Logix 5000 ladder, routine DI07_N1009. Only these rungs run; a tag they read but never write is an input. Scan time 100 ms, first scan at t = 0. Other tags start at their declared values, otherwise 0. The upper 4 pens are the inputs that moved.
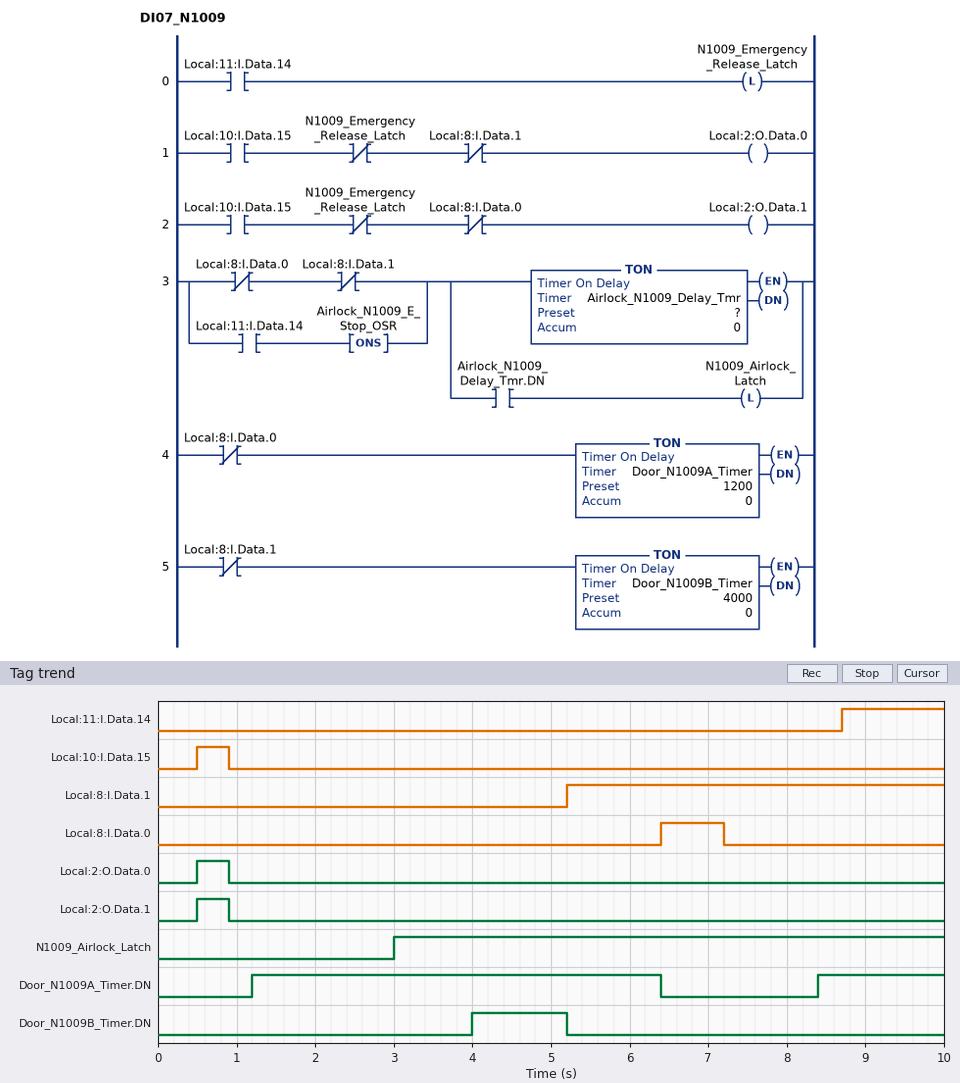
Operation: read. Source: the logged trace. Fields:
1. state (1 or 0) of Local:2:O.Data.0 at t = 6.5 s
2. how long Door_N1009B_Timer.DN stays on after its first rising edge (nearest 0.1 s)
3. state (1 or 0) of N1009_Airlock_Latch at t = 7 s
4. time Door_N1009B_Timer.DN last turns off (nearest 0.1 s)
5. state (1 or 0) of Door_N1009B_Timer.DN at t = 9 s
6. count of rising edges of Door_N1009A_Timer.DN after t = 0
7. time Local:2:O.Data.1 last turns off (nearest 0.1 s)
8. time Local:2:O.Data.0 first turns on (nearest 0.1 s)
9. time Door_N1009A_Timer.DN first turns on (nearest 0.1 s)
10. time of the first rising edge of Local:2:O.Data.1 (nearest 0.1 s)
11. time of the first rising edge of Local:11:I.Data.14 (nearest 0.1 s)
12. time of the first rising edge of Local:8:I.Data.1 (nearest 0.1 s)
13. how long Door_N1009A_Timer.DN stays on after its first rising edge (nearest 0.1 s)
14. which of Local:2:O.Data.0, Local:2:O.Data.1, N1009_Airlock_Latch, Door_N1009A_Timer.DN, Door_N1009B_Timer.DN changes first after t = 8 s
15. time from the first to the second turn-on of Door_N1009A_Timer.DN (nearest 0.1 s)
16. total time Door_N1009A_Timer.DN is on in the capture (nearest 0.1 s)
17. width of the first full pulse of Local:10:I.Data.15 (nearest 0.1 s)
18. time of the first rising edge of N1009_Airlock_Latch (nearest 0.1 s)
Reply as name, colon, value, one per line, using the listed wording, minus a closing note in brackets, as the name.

state (1 or 0) of Local:2:O.Data.0 at t = 6.5 s: 0
how long Door_N1009B_Timer.DN stays on after its first rising edge: 1.2 s
state (1 or 0) of N1009_Airlock_Latch at t = 7 s: 1
time Door_N1009B_Timer.DN last turns off: 5.2 s
state (1 or 0) of Door_N1009B_Timer.DN at t = 9 s: 0
count of rising edges of Door_N1009A_Timer.DN after t = 0: 2
time Local:2:O.Data.1 last turns off: 0.9 s
time Local:2:O.Data.0 first turns on: 0.5 s
time Door_N1009A_Timer.DN first turns on: 1.2 s
time of the first rising edge of Local:2:O.Data.1: 0.5 s
time of the first rising edge of Local:11:I.Data.14: 8.7 s
time of the first rising edge of Local:8:I.Data.1: 5.2 s
how long Door_N1009A_Timer.DN stays on after its first rising edge: 5.2 s
which of Local:2:O.Data.0, Local:2:O.Data.1, N1009_Airlock_Latch, Door_N1009A_Timer.DN, Door_N1009B_Timer.DN changes first after t = 8 s: Door_N1009A_Timer.DN
time from the first to the second turn-on of Door_N1009A_Timer.DN: 7.2 s
total time Door_N1009A_Timer.DN is on in the capture: 6.8 s
width of the first full pulse of Local:10:I.Data.15: 0.4 s
time of the first rising edge of N1009_Airlock_Latch: 3.0 s
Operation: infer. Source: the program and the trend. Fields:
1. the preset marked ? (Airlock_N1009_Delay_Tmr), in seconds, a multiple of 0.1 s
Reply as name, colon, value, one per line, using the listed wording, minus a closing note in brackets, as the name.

the preset marked ? (Airlock_N1009_Delay_Tmr), in seconds, a multiple of 0.1 s: 3.0 s
